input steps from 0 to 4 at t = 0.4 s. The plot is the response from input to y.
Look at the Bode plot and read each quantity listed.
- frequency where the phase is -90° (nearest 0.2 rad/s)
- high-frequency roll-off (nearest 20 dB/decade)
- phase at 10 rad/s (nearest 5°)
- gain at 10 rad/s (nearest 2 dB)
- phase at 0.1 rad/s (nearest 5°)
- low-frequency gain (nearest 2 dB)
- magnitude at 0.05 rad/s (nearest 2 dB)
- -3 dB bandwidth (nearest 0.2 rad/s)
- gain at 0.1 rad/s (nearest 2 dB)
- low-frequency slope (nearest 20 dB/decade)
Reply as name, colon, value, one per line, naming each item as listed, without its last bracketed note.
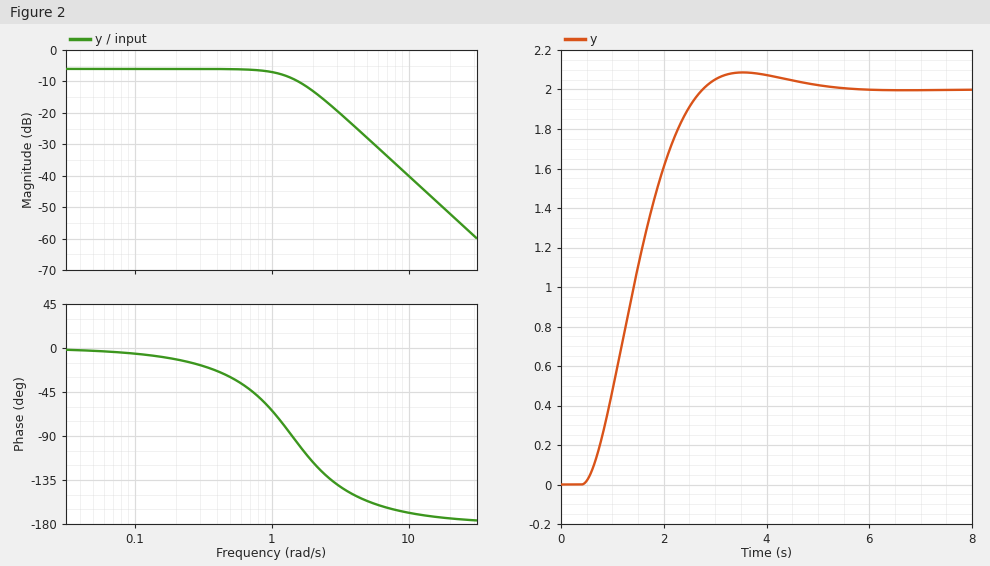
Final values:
frequency where the phase is -90°: 1.4 rad/s
high-frequency roll-off: -40 dB/decade
phase at 10 rad/s: -170°
gain at 10 rad/s: -40 dB
phase at 0.1 rad/s: -5°
low-frequency gain: -6 dB
magnitude at 0.05 rad/s: -6 dB
-3 dB bandwidth: 1.4 rad/s
gain at 0.1 rad/s: -6 dB
low-frequency slope: 0 dB/decade
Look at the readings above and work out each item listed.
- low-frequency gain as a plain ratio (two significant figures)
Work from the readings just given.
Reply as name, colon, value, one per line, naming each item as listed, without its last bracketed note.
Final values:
low-frequency gain as a plain ratio: 0.50
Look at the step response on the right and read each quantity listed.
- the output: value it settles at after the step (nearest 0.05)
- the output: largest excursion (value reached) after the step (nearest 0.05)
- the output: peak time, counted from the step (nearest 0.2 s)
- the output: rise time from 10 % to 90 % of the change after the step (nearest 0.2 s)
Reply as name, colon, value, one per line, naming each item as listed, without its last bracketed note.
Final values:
the output: value it settles at after the step: 2.00
the output: largest excursion (value reached) after the step: 2.10
the output: peak time, counted from the step: 3.2 s
the output: rise time from 10 % to 90 % of the change after the step: 1.6 s
